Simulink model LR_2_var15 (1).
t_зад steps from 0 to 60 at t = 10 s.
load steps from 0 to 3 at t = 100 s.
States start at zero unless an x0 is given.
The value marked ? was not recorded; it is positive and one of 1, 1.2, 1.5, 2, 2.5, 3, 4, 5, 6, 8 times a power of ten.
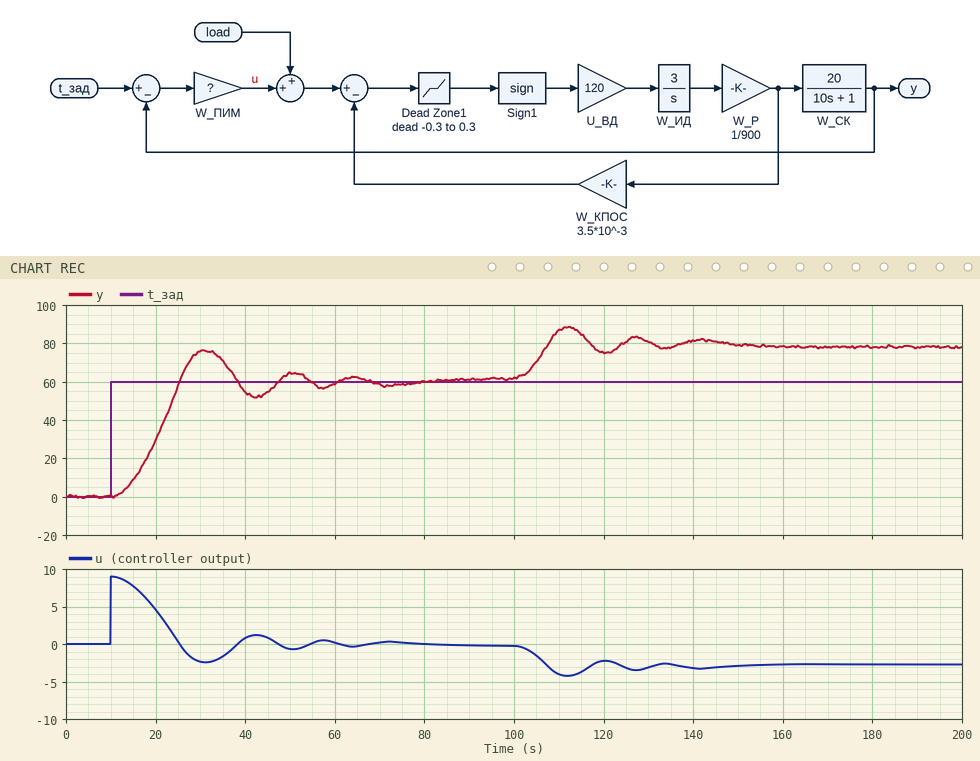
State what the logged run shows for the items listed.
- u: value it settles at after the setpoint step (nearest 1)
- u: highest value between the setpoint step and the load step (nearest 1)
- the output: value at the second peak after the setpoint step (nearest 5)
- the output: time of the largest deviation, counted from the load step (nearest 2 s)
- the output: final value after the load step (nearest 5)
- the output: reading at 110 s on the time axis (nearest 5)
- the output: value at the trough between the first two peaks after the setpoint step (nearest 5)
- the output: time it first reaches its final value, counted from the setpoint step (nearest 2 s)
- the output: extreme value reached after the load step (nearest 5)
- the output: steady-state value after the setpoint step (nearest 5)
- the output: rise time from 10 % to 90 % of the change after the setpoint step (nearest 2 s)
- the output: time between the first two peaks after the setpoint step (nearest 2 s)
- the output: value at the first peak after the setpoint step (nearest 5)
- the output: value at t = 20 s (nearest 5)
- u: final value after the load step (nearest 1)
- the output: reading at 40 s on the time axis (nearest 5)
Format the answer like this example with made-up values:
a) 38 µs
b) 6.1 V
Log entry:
a) 0
b) 9
c) 65
d) 12 s
e) 80
f) 85
g) 50
h) 16 s
i) 90
j) 60
k) 10 s
l) 20 s
m) 75
n) 30
o) -3
p) 55
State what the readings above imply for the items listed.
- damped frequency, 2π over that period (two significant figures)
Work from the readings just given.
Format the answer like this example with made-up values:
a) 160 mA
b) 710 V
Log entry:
a) 0.31 rad/s
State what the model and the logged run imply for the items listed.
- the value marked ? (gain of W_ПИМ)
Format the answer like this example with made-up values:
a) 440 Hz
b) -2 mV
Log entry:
a) 0.15
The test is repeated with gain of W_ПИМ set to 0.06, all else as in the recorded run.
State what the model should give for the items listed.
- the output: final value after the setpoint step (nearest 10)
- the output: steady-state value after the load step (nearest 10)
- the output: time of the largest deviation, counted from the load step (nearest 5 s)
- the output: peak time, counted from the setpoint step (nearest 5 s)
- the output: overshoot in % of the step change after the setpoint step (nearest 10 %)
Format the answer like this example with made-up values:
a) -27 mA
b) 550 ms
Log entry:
a) 60
b) 110
c) 20 s
d) 20 s
e) 30 %
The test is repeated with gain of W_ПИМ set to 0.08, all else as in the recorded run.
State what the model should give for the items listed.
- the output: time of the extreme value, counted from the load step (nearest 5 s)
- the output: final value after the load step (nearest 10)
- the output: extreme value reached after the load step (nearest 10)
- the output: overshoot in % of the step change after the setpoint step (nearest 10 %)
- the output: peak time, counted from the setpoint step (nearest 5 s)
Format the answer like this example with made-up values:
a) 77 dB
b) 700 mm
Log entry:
a) 15 s
b) 100
c) 110
d) 20 %
e) 20 s
